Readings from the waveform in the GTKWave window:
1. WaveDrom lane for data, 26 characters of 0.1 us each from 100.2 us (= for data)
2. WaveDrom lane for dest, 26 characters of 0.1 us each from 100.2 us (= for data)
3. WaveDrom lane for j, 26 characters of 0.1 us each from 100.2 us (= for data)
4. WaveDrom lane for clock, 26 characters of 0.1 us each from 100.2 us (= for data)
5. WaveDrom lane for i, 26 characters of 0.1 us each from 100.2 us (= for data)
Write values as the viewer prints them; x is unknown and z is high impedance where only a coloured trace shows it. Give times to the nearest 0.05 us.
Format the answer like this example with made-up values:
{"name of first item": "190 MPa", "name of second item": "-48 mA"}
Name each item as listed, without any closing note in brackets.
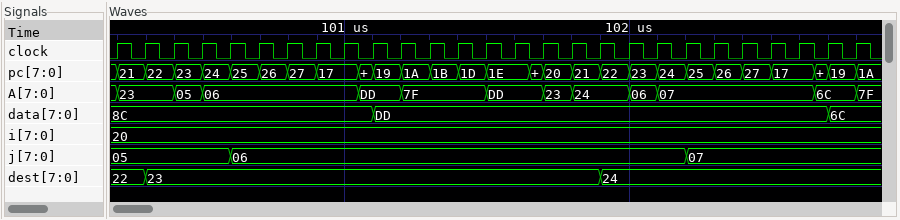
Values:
{"WaveDrom lane for data, 26 characters of 0.1 us each from 100.2 us": "{name: 'data', wave: '=........=...............=', data: '8C DD 6C'}", "WaveDrom lane for dest, 26 characters of 0.1 us each from 100.2 us": "{name: 'dest', wave: '==...............=........', data: '22 23 24'}", "WaveDrom lane for j, 26 characters of 0.1 us each from 100.2 us": "{name: 'j', wave: '=...=...............=.....', data: '05 06 07'}", "WaveDrom lane for clock, 26 characters of 0.1 us each from 100.2 us": "{name: 'clock', wave: 'p.........................'}", "WaveDrom lane for i, 26 characters of 0.1 us each from 100.2 us": "{name: 'i', wave: '=.........................', data: '20'}"}
